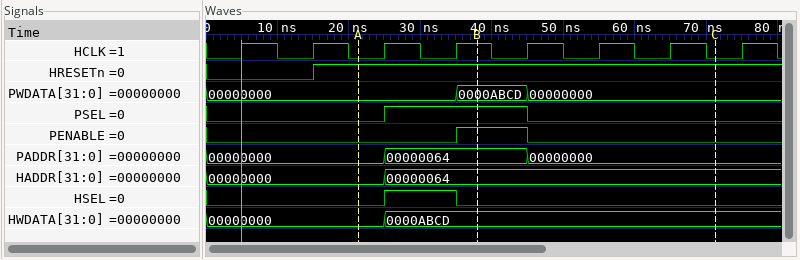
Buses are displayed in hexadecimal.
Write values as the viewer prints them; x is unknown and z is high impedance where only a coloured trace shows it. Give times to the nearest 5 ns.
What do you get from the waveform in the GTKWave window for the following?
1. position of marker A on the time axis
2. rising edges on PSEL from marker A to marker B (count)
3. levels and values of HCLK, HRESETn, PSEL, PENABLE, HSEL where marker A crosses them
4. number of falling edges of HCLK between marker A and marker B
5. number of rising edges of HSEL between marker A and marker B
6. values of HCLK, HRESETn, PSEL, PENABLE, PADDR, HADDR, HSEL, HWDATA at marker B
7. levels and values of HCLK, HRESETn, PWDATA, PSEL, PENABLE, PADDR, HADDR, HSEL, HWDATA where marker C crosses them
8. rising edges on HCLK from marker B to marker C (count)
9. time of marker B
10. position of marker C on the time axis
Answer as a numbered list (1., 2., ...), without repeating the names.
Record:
1. 20 ns
2. 1
3. HCLK=0, HRESETn=1, PSEL=0, PENABLE=0, HSEL=0
4. 1
5. 1
6. HCLK=1, HRESETn=1, PSEL=1, PENABLE=1, PADDR=00000064, HADDR=00000064, HSEL=0, HWDATA=0000ABCD
7. HCLK=0, HRESETn=1, PWDATA=00000000, PSEL=0, PENABLE=0, PADDR=00000000, HADDR=00000064, HSEL=0, HWDATA=0000ABCD
8. 3
9. 40 ns
10. 70 ns
